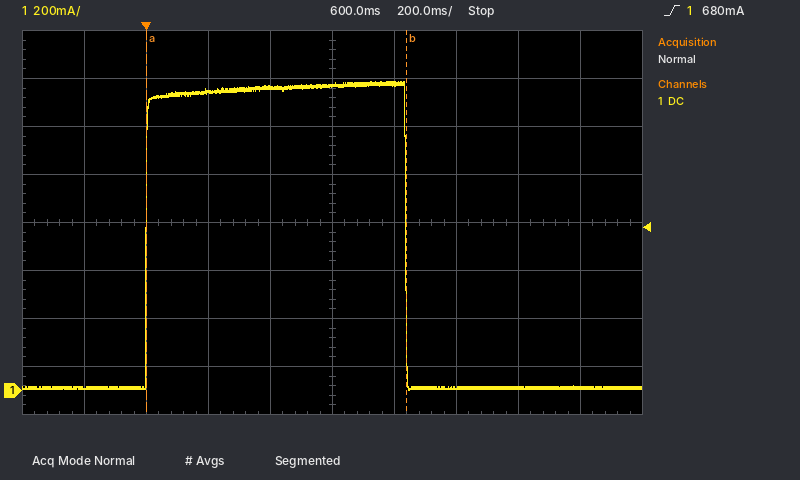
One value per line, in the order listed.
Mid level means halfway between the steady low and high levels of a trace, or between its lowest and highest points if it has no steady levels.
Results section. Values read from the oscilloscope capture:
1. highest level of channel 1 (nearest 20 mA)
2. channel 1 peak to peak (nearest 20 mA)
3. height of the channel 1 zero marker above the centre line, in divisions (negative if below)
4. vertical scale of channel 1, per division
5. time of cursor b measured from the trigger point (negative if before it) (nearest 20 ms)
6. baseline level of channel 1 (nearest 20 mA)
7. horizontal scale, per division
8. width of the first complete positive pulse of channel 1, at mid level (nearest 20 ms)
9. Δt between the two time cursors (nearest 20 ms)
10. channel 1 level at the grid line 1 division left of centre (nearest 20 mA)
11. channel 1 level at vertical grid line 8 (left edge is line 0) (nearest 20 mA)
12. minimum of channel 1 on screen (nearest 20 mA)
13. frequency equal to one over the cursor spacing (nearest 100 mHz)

1.28 A
1.28 A
-3.5 div
200 mA
+840 ms
20 mA
200 ms
840 ms
840 ms
1.26 A
20 mA
0 mA
1.2 Hz
